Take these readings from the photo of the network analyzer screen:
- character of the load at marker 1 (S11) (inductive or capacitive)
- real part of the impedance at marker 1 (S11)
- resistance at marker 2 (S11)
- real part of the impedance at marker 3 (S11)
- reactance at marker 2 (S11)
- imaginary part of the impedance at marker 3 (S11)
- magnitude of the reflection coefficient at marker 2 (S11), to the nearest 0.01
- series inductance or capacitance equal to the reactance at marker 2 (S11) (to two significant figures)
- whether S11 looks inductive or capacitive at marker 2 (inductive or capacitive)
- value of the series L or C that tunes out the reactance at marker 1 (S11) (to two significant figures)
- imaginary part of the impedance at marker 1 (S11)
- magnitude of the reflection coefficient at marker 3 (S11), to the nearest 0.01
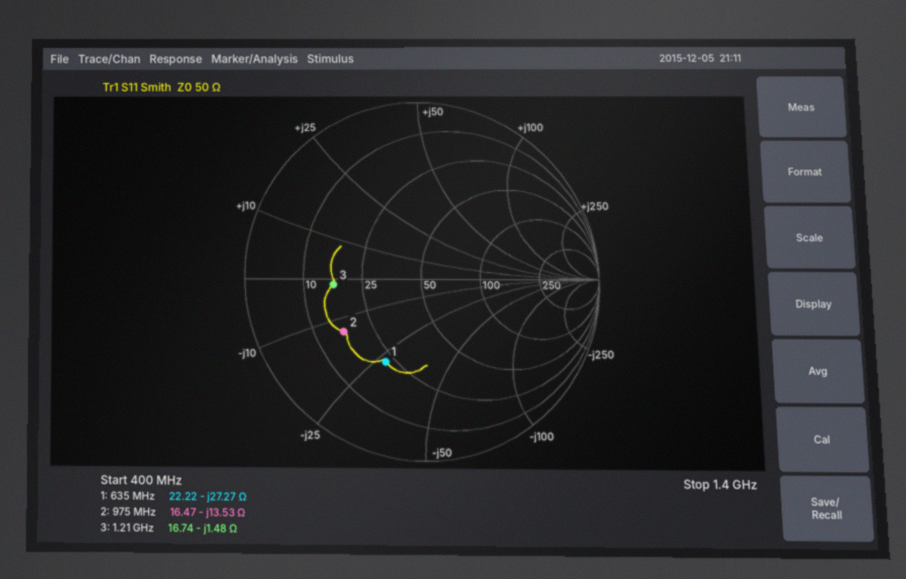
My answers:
capacitive
22.22 Ω
16.47 Ω
16.74 Ω
-13.53 Ω
-1.48 Ω
0.53
12 pF
capacitive
6.8 nH
-27.27 Ω
0.50
